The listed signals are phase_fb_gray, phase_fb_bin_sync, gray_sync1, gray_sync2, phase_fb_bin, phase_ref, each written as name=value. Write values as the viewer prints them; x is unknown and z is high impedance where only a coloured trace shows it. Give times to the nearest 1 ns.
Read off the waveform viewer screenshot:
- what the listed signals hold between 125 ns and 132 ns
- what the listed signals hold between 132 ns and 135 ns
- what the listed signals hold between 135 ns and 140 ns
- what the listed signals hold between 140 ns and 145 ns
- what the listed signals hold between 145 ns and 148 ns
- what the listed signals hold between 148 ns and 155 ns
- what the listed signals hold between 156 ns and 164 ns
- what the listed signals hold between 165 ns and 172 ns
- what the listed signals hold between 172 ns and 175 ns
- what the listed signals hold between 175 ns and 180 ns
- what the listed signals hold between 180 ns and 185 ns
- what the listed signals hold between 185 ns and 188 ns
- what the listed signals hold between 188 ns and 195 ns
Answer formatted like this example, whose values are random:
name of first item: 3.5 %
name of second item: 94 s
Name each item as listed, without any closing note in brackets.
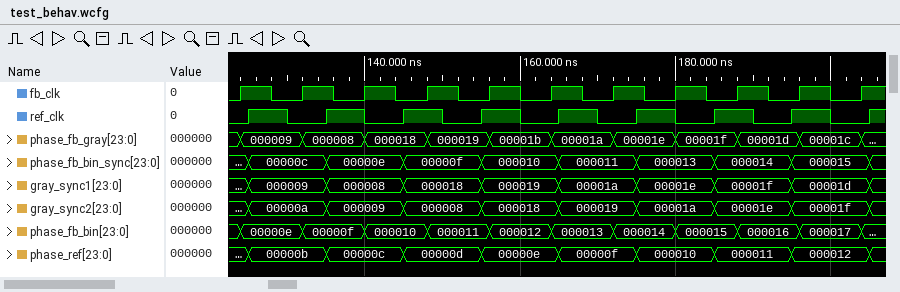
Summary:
what the listed signals hold between 125 ns and 132 ns: phase_fb_gray=000009, phase_fb_bin_sync=00000c, gray_sync1=000009, gray_sync2=00000a, phase_fb_bin=00000e, phase_ref=00000b
what the listed signals hold between 132 ns and 135 ns: phase_fb_gray=000008, phase_fb_bin_sync=00000c, gray_sync1=000009, gray_sync2=00000a, phase_fb_bin=00000f, phase_ref=00000b
what the listed signals hold between 135 ns and 140 ns: phase_fb_gray=000008, phase_fb_bin_sync=00000e, gray_sync1=000008, gray_sync2=000009, phase_fb_bin=00000f, phase_ref=00000c
what the listed signals hold between 140 ns and 145 ns: phase_fb_gray=000018, phase_fb_bin_sync=00000e, gray_sync1=000008, gray_sync2=000009, phase_fb_bin=000010, phase_ref=00000c
what the listed signals hold between 145 ns and 148 ns: phase_fb_gray=000018, phase_fb_bin_sync=00000f, gray_sync1=000018, gray_sync2=000008, phase_fb_bin=000010, phase_ref=00000d
what the listed signals hold between 148 ns and 155 ns: phase_fb_gray=000019, phase_fb_bin_sync=00000f, gray_sync1=000018, gray_sync2=000008, phase_fb_bin=000011, phase_ref=00000d
what the listed signals hold between 156 ns and 164 ns: phase_fb_gray=00001b, phase_fb_bin_sync=000010, gray_sync1=000019, gray_sync2=000018, phase_fb_bin=000012, phase_ref=00000e
what the listed signals hold between 165 ns and 172 ns: phase_fb_gray=00001a, phase_fb_bin_sync=000011, gray_sync1=00001a, gray_sync2=000019, phase_fb_bin=000013, phase_ref=00000f
what the listed signals hold between 172 ns and 175 ns: phase_fb_gray=00001e, phase_fb_bin_sync=000011, gray_sync1=00001a, gray_sync2=000019, phase_fb_bin=000014, phase_ref=00000f
what the listed signals hold between 175 ns and 180 ns: phase_fb_gray=00001e, phase_fb_bin_sync=000013, gray_sync1=00001e, gray_sync2=00001a, phase_fb_bin=000014, phase_ref=000010
what the listed signals hold between 180 ns and 185 ns: phase_fb_gray=00001f, phase_fb_bin_sync=000013, gray_sync1=00001e, gray_sync2=00001a, phase_fb_bin=000015, phase_ref=000010
what the listed signals hold between 185 ns and 188 ns: phase_fb_gray=00001f, phase_fb_bin_sync=000014, gray_sync1=00001f, gray_sync2=00001e, phase_fb_bin=000015, phase_ref=000011
what the listed signals hold between 188 ns and 195 ns: phase_fb_gray=00001d, phase_fb_bin_sync=000014, gray_sync1=00001f, gray_sync2=00001e, phase_fb_bin=000016, phase_ref=000011
